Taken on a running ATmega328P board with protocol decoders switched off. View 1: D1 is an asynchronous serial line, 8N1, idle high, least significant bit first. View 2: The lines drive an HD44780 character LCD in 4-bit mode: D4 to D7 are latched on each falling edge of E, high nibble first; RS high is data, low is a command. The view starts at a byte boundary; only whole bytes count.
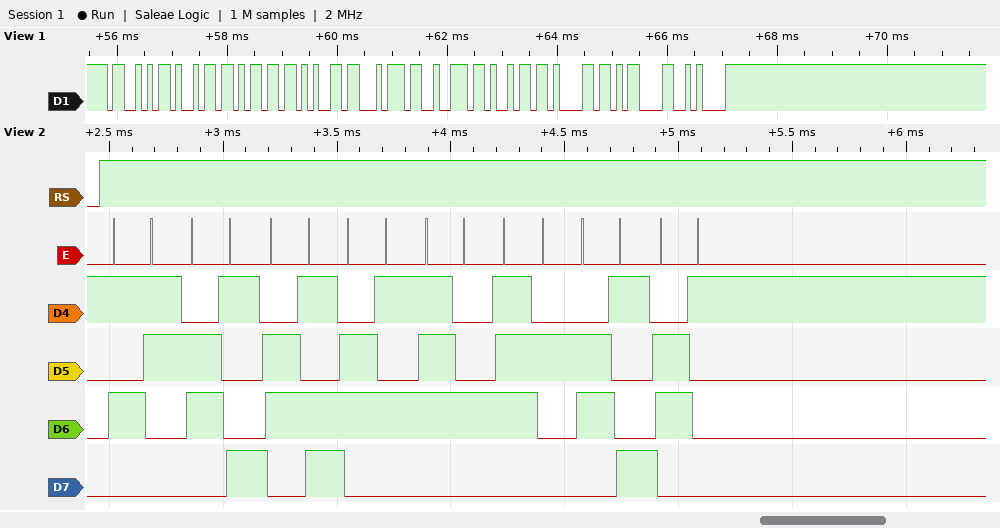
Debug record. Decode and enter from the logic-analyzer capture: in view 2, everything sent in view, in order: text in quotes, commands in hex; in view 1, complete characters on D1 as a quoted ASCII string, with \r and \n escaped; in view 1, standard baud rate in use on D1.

"Simetria"
"Simetria\r\n"
9600 baud
